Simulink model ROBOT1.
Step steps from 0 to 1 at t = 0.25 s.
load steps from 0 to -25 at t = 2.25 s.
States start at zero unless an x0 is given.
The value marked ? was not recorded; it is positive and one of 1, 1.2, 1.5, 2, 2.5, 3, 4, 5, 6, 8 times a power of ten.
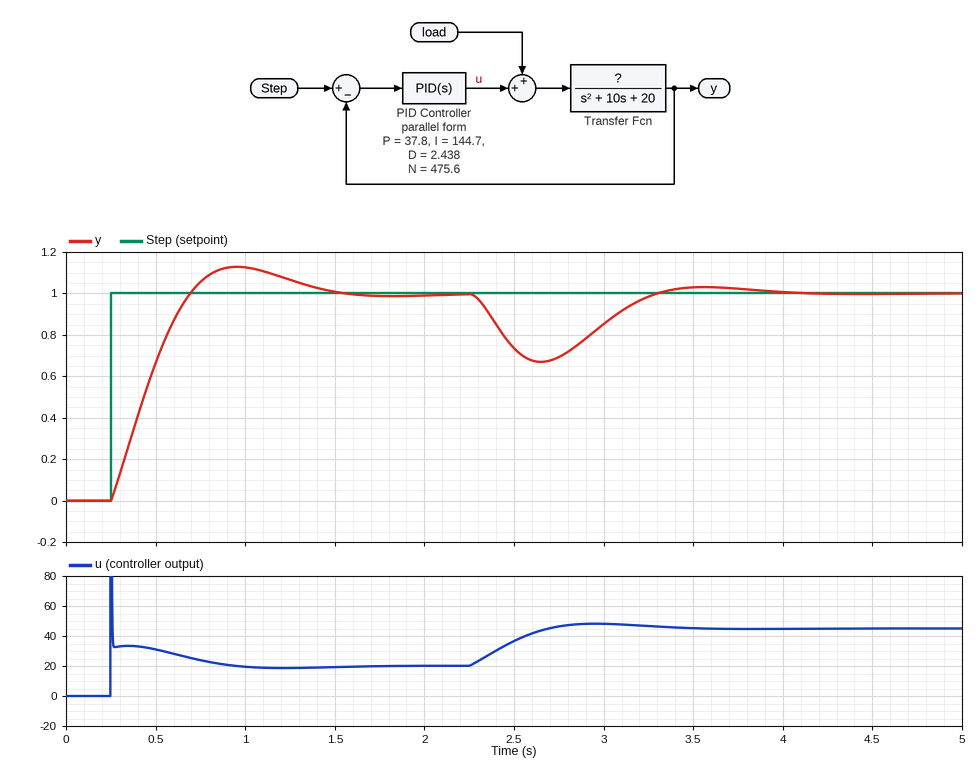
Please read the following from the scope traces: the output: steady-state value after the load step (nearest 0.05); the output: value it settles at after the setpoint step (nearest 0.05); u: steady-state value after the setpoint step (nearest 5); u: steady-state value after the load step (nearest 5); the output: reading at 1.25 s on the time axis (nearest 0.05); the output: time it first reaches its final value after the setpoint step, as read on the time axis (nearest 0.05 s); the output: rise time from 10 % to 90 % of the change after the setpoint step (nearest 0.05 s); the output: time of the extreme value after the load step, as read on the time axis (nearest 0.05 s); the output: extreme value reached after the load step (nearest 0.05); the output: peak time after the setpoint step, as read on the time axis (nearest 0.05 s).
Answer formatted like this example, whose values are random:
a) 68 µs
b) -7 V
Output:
a) 1.00
b) 1.00
c) 20
d) 45
e) 1.05
f) 0.70 s
g) 0.35 s
h) 2.65 s
i) 0.65
j) 0.95 s
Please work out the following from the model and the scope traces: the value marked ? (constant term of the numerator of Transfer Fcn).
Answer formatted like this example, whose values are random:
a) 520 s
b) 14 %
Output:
a) 1
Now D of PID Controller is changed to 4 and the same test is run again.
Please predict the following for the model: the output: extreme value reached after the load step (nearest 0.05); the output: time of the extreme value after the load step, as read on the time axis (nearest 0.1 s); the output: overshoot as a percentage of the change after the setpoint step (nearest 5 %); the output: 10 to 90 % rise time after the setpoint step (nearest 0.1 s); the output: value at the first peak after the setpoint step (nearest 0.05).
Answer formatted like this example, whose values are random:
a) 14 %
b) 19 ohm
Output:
a) 0.70
b) 2.7 s
c) 10 %
d) 0.4 s
e) 1.10
